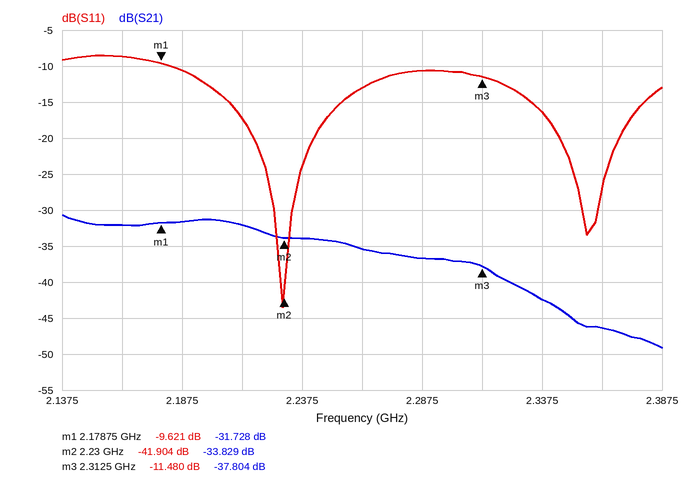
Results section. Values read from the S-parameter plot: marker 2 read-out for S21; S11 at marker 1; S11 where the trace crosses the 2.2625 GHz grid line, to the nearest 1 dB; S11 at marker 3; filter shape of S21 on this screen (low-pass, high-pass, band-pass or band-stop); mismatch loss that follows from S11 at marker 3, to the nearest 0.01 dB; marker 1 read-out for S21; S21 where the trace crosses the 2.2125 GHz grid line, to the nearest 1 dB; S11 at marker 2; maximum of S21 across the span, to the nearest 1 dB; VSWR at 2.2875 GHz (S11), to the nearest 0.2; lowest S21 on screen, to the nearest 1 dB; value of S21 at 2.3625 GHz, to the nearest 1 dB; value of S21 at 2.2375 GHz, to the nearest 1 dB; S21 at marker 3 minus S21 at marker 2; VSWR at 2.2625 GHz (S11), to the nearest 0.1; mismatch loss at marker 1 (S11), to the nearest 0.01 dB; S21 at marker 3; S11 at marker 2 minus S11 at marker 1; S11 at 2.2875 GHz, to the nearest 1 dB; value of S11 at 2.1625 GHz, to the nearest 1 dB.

-33.829 dB
-9.621 dB
-13 dB
-11.480 dB
low-pass
0.32 dB
-31.728 dB
-32 dB
-41.904 dB
-31 dB
1.8
-49 dB
-46 dB
-34 dB
-3.975 dB
1.6
0.50 dB
-37.804 dB
-32.283 dB
-11 dB
-9 dB
